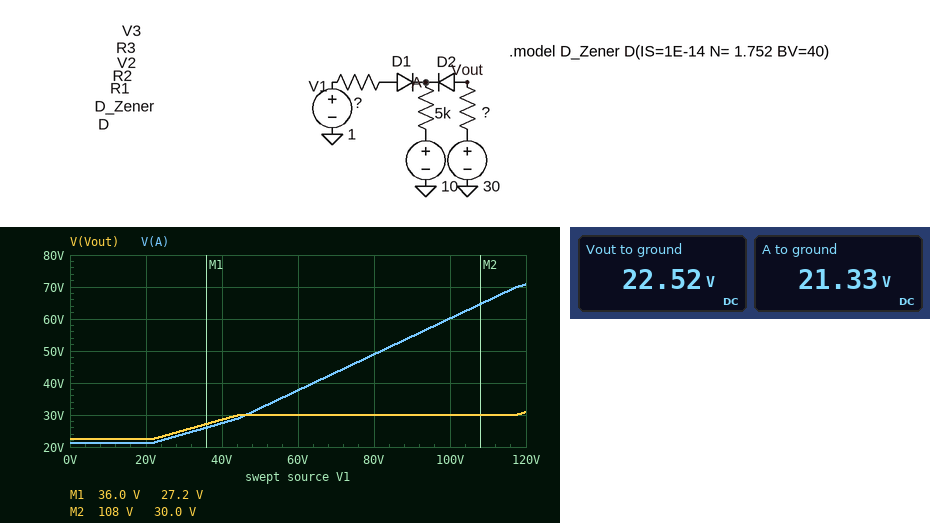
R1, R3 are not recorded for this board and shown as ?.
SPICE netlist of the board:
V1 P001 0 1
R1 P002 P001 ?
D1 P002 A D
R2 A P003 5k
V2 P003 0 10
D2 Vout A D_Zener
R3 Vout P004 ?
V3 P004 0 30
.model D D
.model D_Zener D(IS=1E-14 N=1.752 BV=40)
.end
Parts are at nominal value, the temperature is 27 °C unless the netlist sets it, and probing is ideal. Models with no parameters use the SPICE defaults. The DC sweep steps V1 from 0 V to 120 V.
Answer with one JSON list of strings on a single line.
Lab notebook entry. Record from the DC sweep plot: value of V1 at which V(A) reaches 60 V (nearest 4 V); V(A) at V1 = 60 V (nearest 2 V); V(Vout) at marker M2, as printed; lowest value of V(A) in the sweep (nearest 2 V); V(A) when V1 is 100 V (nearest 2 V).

["100 V", "38 V", "30.0 V", "22 V", "60 V"]
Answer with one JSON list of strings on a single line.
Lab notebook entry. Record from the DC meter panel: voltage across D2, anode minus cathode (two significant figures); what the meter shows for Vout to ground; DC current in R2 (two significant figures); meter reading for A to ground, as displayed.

["1.2 V", "22.52 V", "2.3 mA", "21.33 V"]
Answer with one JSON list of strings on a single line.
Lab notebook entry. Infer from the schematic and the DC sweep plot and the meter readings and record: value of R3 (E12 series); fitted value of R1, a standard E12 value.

["3.3 kΩ", "3.9 kΩ"]
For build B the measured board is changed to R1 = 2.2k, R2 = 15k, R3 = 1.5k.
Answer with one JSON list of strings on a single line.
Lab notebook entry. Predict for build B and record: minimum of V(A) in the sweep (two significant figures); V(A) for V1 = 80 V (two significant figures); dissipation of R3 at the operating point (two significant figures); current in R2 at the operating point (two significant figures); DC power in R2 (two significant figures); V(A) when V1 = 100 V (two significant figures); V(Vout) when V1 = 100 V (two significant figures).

["27 V", "70 V", "2.0 mW", "1.1 mA", "20 mW", "78 V", "38 V"]
